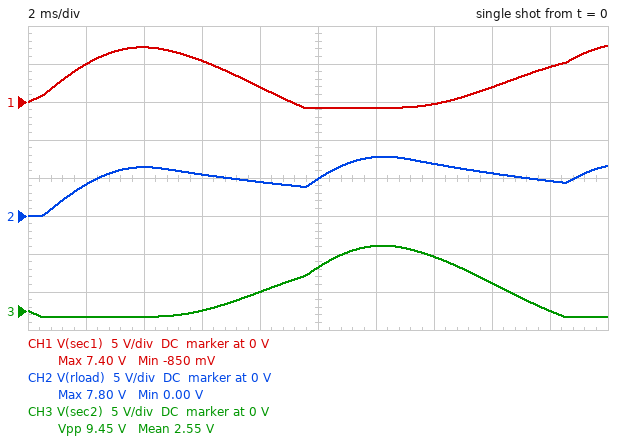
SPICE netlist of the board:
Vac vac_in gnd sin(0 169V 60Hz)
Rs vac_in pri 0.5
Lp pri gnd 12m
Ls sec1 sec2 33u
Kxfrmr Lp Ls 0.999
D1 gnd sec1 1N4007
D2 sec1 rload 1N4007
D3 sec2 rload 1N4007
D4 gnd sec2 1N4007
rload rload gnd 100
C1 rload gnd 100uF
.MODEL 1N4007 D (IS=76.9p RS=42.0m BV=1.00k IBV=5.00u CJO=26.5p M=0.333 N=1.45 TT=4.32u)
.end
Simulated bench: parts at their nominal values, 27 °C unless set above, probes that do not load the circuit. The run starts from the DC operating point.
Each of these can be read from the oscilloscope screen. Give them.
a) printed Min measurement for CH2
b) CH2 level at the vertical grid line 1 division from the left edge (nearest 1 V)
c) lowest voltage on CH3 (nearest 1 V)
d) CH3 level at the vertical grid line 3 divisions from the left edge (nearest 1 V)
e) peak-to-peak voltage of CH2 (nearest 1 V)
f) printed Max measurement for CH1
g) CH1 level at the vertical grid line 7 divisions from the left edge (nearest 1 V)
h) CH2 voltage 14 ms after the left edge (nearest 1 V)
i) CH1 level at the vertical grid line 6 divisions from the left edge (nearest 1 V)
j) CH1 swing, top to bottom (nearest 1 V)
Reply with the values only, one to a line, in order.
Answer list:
0.00 V
4 V
-1 V
0 V
8 V
7.40 V
0 V
7 V
-1 V
8 V
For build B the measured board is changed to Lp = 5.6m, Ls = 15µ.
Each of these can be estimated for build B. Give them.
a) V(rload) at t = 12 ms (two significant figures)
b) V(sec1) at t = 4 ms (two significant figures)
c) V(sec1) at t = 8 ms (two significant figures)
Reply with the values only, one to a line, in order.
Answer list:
7.6 V
6.3 V
940 mV
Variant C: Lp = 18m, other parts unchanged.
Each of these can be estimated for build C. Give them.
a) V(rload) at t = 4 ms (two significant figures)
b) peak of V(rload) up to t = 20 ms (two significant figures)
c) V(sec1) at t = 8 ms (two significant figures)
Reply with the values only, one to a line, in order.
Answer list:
5.2 V
6.0 V
1.8 V
